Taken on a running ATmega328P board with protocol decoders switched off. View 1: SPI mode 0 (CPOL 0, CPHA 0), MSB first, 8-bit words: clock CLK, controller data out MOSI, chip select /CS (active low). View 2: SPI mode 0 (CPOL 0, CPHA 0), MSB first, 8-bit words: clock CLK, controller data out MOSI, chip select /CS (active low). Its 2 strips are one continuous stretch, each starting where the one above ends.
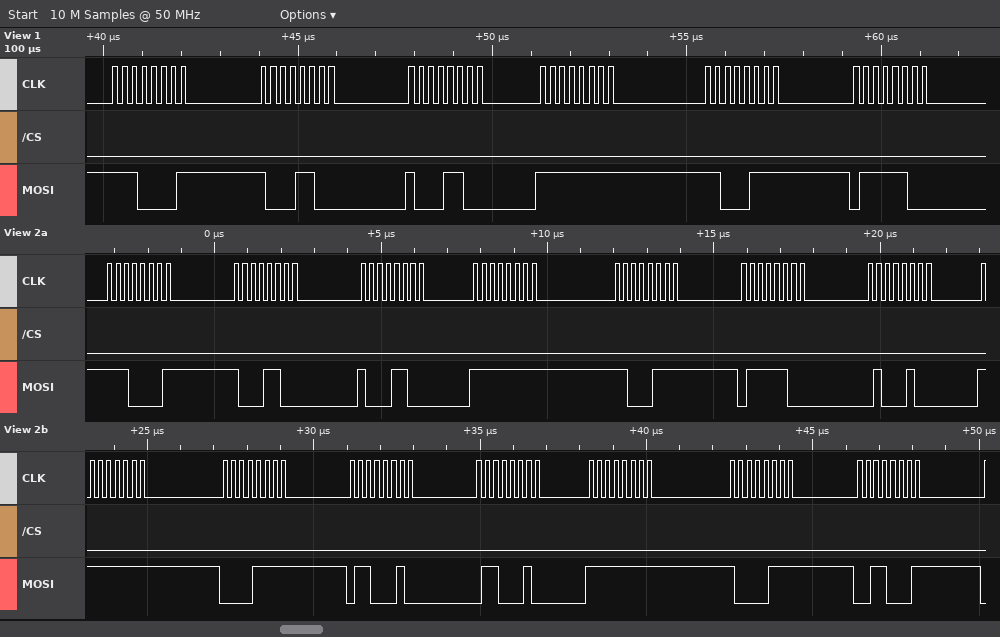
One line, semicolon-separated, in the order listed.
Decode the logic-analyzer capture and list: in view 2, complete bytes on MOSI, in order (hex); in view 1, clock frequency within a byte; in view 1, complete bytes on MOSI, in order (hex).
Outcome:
E1 8C 8C FF C7 7C 44 FF 0F 62 62 FF 87 31; 4 MHz; 0xE1 0x8C 0x8C 0xFF 0xC7 0x7C
